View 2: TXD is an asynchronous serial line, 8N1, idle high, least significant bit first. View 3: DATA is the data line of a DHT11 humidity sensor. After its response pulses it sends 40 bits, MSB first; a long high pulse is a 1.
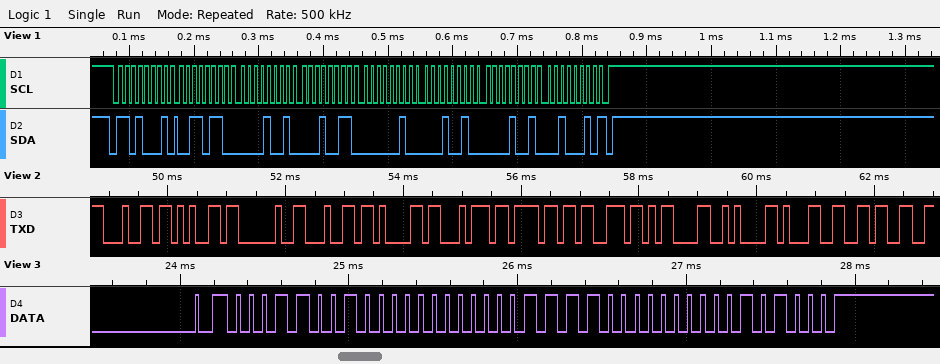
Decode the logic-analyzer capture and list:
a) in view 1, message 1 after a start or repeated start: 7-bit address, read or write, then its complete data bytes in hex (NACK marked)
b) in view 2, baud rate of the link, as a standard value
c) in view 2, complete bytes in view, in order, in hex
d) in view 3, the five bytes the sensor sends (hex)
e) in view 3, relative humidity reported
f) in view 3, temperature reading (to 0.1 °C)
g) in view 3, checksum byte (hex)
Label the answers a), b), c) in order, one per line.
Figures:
a) 0x68 read: 36 09 13 02 12 09 22 NACK
b) 9600 baud
c) 0x64 0x65 0x20 0x64 0x61 0x74 0x6F 0x73 0x0D 0x0A 0x31 0x36
d) 19 00 0F 00 28
e) 25 %
f) 15.0 °C
g) 0x28
